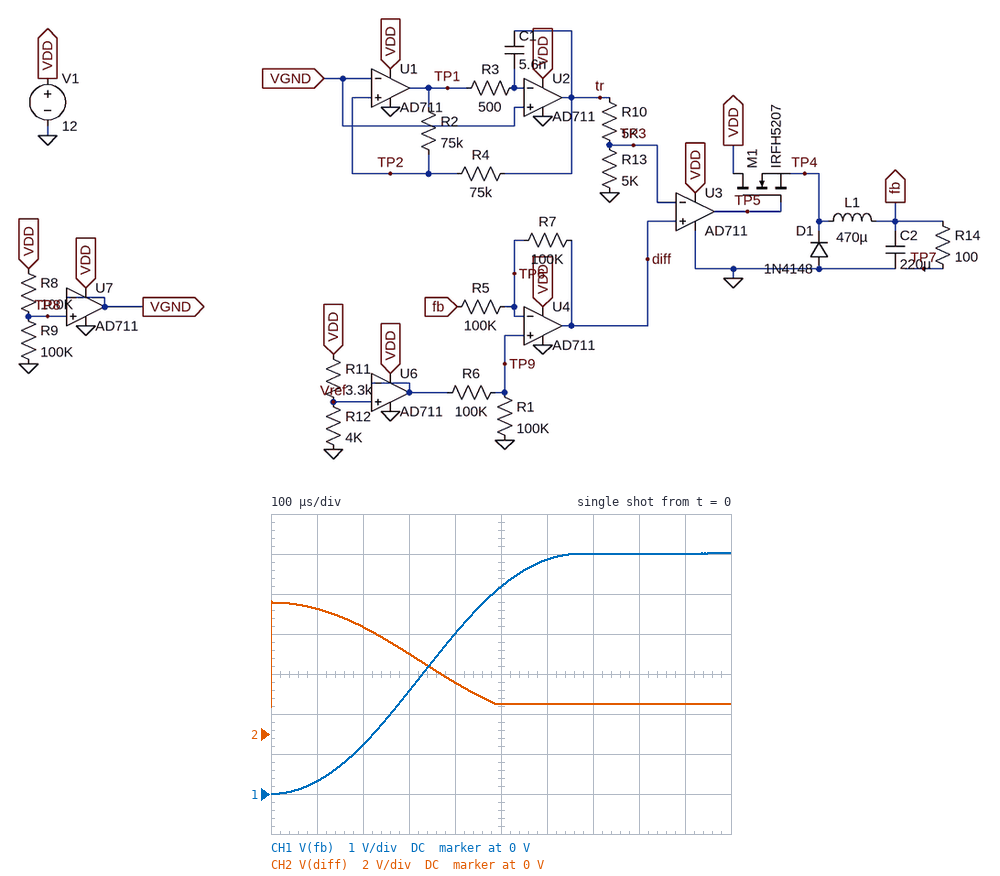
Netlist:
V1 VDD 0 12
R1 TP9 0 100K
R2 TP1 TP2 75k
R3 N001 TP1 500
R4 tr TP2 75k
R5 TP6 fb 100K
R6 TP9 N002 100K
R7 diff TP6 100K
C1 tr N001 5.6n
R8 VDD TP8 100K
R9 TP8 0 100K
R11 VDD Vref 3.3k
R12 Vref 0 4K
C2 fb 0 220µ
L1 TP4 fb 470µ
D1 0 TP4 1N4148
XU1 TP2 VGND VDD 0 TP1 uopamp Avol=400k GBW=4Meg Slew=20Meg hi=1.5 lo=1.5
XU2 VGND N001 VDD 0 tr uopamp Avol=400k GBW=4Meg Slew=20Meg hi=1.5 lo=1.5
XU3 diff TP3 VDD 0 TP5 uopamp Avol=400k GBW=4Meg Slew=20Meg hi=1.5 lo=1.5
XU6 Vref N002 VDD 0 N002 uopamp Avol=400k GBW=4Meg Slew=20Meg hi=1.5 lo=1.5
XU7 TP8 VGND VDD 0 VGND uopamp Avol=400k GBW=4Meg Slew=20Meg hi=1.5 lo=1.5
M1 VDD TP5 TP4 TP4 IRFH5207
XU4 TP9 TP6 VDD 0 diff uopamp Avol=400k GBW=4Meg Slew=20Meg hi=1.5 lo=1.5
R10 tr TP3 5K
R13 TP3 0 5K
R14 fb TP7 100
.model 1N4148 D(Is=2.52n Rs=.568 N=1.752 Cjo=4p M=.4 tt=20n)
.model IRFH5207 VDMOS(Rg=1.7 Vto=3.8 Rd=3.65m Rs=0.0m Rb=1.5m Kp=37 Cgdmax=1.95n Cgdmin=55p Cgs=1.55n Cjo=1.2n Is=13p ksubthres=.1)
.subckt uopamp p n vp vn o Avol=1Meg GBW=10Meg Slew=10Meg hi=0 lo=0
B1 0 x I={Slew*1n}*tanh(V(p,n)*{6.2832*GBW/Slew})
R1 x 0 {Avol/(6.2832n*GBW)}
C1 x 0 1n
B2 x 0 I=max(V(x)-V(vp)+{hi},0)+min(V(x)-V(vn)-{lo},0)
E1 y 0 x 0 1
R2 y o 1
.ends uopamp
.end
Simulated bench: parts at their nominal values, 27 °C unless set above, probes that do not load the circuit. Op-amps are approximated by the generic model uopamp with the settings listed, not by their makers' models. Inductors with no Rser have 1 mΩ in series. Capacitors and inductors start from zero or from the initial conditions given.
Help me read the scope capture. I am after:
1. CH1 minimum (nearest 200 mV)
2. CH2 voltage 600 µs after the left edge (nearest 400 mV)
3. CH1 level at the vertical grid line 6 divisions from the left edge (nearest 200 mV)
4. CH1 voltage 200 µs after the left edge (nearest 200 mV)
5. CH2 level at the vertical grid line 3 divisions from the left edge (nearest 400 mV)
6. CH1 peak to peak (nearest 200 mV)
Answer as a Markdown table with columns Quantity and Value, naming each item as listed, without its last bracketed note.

| Quantity | Value |
|---|---|
| CH1 minimum | 0 V |
| CH2 voltage 600 µs after the left edge | 1.6 V |
| CH1 level at the vertical grid line 6 divisions from the left edge | 5.8 V |
| CH1 voltage 200 µs after the left edge | 1.2 V |
| CH2 level at the vertical grid line 3 divisions from the left edge | 4.0 V |
| CH1 peak to peak | 6.0 V |
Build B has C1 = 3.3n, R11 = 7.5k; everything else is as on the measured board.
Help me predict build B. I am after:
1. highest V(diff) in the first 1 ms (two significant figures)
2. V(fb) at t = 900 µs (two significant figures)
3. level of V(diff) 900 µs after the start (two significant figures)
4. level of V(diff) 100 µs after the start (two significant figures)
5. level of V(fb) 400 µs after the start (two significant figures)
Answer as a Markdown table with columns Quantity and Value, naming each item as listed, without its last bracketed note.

| Quantity | Value |
|---|---|
| highest V(diff) in the first 1 ms | 4.2 V |
| V(fb) at t = 900 µs | 3.4 V |
| level of V(diff) 900 µs after the start | 1.5 V |
| level of V(diff) 100 µs after the start | 4.0 V |
| level of V(fb) 400 µs after the start | 2.2 V |
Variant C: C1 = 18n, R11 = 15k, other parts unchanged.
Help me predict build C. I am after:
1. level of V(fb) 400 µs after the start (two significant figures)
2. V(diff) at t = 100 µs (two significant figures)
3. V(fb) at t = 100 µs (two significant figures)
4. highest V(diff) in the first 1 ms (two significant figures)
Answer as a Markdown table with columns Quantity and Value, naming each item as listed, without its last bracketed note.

| Quantity | Value |
|---|---|
| level of V(fb) 400 µs after the start | 1.0 V |
| V(diff) at t = 100 µs | 2.4 V |
| V(fb) at t = 100 µs | 85 mV |
| highest V(diff) in the first 1 ms | 2.5 V |
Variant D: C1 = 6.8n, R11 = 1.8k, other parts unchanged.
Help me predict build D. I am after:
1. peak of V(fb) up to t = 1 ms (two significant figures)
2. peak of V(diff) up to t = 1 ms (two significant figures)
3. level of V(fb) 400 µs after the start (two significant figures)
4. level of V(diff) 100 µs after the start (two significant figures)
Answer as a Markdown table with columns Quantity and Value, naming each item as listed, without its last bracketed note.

| Quantity | Value |
|---|---|
| peak of V(fb) up to t = 1 ms | 7.6 V |
| peak of V(diff) up to t = 1 ms | 8.3 V |
| level of V(fb) 400 µs after the start | 4.3 V |
| level of V(diff) 100 µs after the start | 8.0 V |
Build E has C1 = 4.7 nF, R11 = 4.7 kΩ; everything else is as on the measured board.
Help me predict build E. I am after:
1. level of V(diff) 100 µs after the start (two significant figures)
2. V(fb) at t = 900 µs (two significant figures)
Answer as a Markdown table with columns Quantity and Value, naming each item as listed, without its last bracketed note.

| Quantity | Value |
|---|---|
| level of V(diff) 100 µs after the start | 5.2 V |
| V(fb) at t = 900 µs | 4.9 V |
